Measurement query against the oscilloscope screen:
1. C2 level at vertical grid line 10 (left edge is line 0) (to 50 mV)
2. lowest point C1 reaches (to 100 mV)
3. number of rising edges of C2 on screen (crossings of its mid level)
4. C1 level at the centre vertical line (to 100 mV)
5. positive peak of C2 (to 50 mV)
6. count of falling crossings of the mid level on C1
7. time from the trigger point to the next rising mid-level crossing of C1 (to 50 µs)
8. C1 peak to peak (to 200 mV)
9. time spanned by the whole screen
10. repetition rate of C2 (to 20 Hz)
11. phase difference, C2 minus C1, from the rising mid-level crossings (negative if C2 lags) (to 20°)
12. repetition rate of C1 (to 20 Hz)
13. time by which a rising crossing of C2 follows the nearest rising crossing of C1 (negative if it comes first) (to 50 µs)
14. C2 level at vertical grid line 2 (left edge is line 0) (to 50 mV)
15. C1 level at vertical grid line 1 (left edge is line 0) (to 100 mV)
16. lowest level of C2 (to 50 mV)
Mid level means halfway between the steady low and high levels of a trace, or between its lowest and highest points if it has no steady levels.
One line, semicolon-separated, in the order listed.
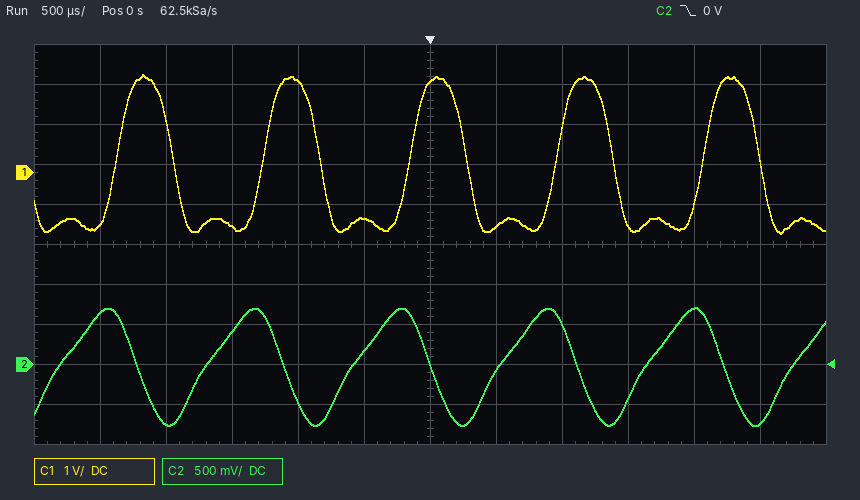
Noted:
700 mV; -1.5 V; 6; 2.3 V; 700 mV; 5; 950 µs; 4.0 V; 6 ms; 900 Hz; +140°; 900 Hz; -450 µs; -750 mV; -1.3 V; -750 mV
